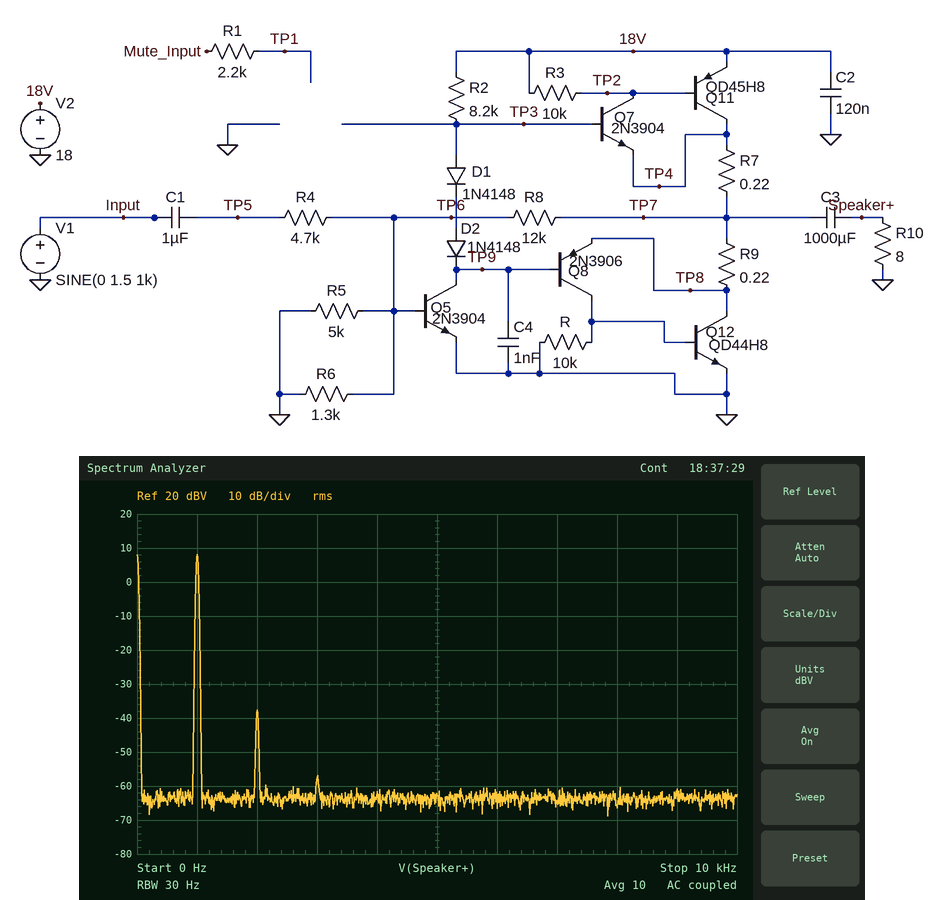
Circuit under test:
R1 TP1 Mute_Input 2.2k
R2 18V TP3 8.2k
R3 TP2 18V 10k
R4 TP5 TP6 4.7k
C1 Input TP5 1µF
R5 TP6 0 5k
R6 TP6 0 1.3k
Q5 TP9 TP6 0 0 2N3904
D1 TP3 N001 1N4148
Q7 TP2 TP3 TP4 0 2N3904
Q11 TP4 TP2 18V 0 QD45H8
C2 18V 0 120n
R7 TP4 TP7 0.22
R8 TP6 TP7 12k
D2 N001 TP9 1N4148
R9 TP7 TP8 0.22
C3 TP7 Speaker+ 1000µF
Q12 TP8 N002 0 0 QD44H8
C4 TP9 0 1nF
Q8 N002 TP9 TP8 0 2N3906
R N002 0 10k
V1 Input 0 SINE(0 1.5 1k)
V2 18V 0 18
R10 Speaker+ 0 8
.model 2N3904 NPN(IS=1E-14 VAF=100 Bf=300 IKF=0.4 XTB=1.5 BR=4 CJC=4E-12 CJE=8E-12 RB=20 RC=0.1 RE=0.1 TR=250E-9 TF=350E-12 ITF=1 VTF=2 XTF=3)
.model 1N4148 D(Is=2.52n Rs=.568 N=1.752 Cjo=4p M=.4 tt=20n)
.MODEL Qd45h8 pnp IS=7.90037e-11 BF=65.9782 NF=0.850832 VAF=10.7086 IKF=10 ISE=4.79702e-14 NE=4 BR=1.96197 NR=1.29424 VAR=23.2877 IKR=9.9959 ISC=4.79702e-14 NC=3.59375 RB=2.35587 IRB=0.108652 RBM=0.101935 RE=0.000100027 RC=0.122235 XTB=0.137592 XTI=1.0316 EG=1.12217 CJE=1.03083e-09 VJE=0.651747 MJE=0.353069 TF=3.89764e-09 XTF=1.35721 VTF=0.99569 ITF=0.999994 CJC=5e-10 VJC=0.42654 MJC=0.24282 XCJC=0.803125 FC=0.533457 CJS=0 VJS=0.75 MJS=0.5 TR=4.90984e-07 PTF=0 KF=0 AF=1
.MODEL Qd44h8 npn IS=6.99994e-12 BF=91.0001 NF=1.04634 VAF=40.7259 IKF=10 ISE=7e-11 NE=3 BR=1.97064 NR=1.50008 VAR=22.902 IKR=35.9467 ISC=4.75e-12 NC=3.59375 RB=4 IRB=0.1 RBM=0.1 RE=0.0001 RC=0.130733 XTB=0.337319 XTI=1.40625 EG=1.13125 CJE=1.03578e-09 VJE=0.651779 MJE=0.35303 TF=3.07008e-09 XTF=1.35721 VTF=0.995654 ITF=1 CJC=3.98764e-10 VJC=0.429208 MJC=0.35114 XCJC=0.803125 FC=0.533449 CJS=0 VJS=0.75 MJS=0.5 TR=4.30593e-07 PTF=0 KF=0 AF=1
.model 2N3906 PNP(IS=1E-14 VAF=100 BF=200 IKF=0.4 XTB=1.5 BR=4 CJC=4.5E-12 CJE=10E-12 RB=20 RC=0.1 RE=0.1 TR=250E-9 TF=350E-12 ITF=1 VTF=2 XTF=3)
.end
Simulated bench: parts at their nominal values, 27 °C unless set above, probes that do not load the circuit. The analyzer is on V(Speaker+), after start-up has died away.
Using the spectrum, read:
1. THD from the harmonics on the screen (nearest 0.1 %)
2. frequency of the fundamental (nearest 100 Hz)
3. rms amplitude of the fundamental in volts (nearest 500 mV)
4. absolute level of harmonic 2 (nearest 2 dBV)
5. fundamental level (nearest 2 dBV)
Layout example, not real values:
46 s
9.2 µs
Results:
0.5 %
1.0 kHz
2.5 V
-38 dBV
8 dBV
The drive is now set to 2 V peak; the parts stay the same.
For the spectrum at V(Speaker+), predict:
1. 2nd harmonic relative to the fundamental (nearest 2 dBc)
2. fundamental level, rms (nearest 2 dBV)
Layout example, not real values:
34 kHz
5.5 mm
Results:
-42 dBc
10 dBV
